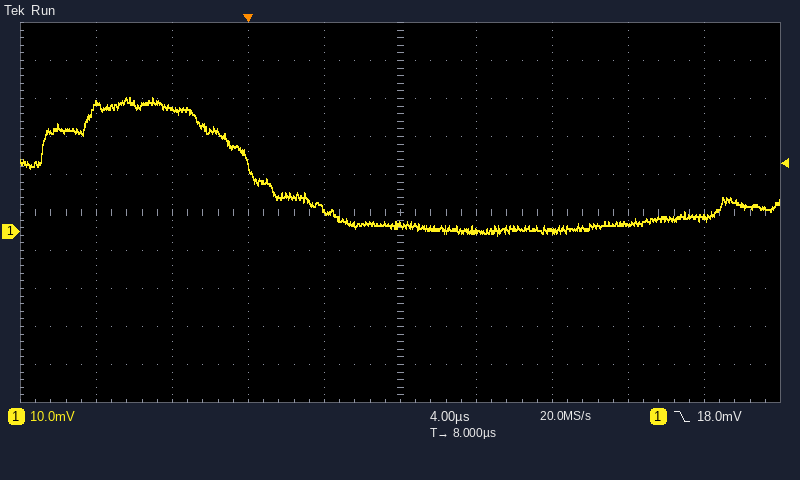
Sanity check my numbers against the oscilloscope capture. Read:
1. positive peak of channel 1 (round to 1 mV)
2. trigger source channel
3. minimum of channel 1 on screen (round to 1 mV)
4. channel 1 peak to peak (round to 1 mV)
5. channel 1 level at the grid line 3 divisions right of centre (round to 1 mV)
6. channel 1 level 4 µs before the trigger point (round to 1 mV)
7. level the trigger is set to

35 mV
channel 1
-1 mV
36 mV
2 mV
32 mV
18.0 mV
